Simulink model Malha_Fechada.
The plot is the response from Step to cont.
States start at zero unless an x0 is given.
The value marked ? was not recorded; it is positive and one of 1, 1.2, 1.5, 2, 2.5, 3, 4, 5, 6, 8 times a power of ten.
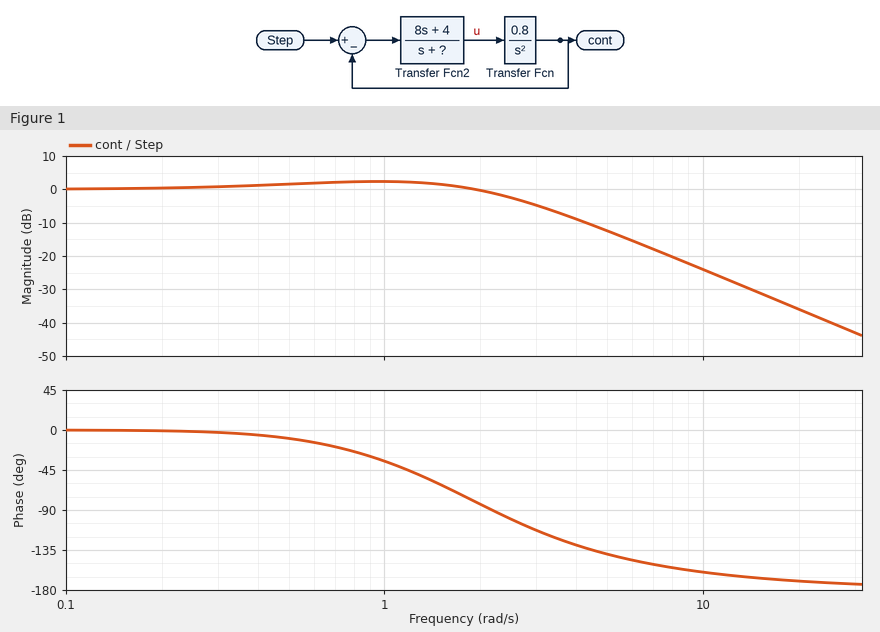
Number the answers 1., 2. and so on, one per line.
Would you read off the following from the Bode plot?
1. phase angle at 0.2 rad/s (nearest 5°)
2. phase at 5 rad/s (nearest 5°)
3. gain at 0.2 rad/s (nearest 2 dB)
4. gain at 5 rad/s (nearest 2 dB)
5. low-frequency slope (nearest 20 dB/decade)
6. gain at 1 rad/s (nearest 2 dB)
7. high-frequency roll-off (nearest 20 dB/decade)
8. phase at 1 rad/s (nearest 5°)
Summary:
1. 0°
2. -140°
3. 0 dB
4. -12 dB
5. 0 dB/decade
6. 2 dB
7. -40 dB/decade
8. -35°
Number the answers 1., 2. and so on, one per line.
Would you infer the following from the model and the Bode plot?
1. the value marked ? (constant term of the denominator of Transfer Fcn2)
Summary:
1. 4
